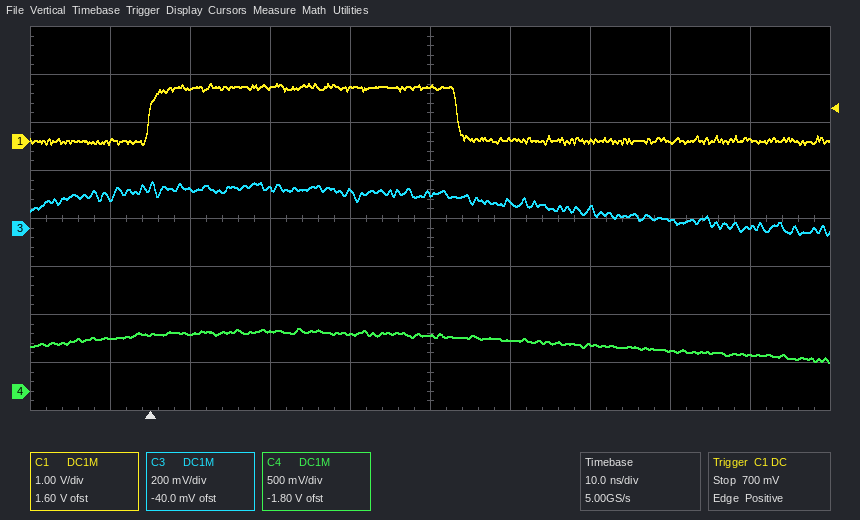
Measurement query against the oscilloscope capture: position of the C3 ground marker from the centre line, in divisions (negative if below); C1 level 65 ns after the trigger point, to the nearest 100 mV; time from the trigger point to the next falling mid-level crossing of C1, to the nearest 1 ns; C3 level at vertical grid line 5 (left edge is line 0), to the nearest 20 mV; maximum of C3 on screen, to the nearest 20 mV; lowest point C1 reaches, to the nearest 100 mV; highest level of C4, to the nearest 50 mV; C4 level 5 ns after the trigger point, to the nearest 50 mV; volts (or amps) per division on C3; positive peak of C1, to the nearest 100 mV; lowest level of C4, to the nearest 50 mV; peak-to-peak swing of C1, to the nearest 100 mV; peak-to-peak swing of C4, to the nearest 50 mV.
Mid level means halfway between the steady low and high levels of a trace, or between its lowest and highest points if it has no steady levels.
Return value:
-0.2 div
0.0 V
38 ns
140 mV
200 mV
-100 mV
650 mV
600 mV
200 mV
1.2 V
300 mV
1.3 V
350 mV
